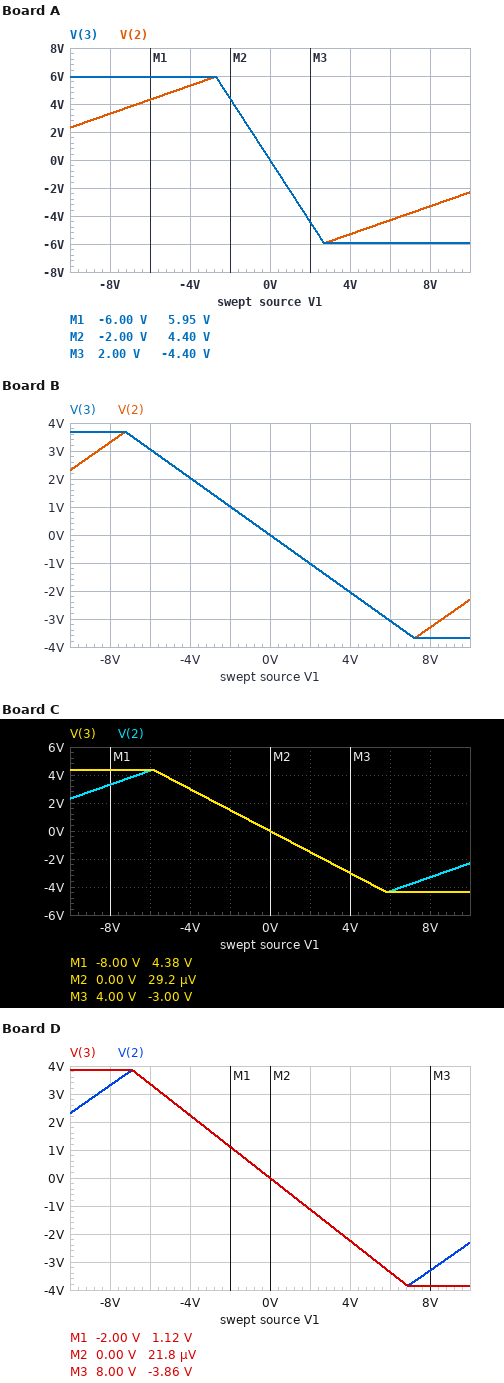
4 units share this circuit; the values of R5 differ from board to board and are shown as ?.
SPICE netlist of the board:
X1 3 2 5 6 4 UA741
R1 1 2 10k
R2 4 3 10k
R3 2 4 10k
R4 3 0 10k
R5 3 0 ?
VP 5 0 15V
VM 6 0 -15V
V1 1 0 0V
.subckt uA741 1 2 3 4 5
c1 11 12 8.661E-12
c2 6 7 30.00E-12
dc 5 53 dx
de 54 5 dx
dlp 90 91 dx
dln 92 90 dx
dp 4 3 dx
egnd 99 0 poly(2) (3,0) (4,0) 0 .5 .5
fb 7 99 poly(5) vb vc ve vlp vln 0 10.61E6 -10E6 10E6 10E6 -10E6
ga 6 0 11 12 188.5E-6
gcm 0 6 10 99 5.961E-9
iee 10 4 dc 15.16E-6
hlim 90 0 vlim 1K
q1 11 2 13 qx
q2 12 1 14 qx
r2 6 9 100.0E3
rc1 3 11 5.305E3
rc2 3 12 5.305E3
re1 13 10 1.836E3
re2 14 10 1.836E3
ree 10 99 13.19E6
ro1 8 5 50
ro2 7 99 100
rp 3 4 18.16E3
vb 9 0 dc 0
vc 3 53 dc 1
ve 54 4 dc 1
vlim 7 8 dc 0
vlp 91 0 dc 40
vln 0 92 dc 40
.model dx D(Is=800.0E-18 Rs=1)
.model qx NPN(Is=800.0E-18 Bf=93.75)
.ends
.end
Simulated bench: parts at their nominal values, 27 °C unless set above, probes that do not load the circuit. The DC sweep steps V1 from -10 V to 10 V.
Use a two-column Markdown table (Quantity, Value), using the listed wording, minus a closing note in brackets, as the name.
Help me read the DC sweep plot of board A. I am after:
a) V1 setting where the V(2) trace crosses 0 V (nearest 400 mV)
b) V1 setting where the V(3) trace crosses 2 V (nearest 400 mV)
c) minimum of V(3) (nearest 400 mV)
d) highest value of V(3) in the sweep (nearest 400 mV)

| Quantity | Value |
|---|---|
| V1 setting where the V(2) trace crosses 0 V | 0 V |
| V1 setting where the V(3) trace crosses 2 V | -800 mV |
| minimum of V(3) | -6.0 V |
| highest value of V(3) in the sweep | 6.0 V |
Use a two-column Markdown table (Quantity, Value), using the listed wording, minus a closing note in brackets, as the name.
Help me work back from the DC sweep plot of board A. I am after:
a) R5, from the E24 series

| Quantity | Value |
|---|---|
| R5, from the E24 series | 22 kΩ |
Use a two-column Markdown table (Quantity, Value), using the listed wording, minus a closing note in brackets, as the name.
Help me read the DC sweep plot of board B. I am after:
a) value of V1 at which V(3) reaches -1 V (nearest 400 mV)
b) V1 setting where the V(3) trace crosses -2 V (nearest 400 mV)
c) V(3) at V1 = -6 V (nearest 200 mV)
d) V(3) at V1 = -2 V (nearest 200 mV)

| Quantity | Value |
|---|---|
| value of V1 at which V(3) reaches -1 V | 2.0 V |
| V1 setting where the V(3) trace crosses -2 V | 4.0 V |
| V(3) at V1 = -6 V | 3.0 V |
| V(3) at V1 = -2 V | 1.0 V |
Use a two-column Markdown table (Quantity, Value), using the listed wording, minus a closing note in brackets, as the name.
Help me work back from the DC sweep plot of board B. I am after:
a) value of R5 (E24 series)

| Quantity | Value |
|---|---|
| value of R5 | 5.1 kΩ |
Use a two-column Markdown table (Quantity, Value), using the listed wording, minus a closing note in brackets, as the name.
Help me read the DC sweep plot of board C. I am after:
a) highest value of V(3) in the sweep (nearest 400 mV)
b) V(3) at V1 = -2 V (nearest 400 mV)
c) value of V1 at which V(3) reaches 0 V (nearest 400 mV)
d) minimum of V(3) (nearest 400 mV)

| Quantity | Value |
|---|---|
| highest value of V(3) in the sweep | 4.4 V |
| V(3) at V1 = -2 V | 1.6 V |
| value of V1 at which V(3) reaches 0 V | 0 V |
| minimum of V(3) | -4.4 V |
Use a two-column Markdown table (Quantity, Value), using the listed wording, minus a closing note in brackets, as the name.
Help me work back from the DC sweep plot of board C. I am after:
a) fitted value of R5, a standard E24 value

| Quantity | Value |
|---|---|
| fitted value of R5, a standard E24 value | 7.5 kΩ |
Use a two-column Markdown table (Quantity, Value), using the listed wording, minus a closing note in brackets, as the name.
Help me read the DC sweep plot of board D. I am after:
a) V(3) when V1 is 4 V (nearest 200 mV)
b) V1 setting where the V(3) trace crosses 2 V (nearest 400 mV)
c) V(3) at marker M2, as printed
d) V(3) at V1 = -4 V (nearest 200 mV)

| Quantity | Value |
|---|---|
| V(3) when V1 is 4 V | -2.2 V |
| V1 setting where the V(3) trace crosses 2 V | -3.6 V |
| V(3) at marker M2, as printed | 21.8 µV |
| V(3) at V1 = -4 V | 2.2 V |
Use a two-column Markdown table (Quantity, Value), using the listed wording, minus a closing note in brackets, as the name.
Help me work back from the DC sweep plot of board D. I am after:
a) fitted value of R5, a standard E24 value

| Quantity | Value |
|---|---|
| fitted value of R5, a standard E24 value | 5.6 kΩ |
